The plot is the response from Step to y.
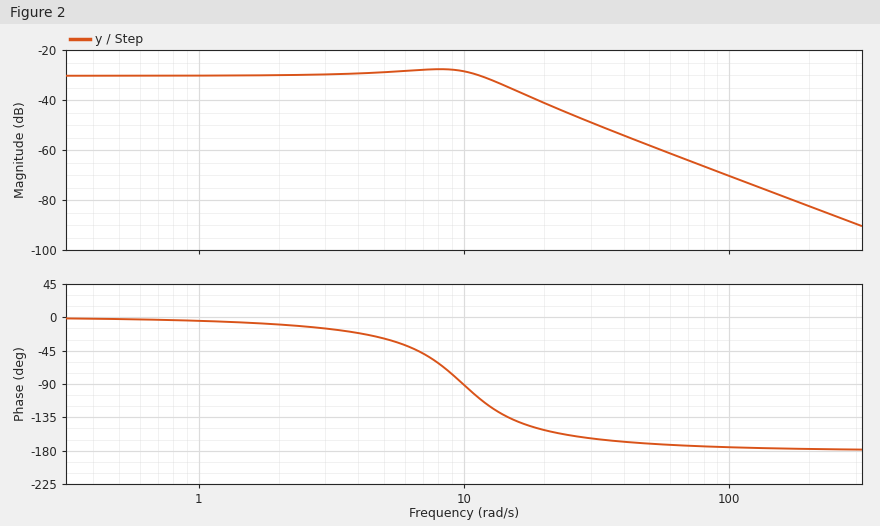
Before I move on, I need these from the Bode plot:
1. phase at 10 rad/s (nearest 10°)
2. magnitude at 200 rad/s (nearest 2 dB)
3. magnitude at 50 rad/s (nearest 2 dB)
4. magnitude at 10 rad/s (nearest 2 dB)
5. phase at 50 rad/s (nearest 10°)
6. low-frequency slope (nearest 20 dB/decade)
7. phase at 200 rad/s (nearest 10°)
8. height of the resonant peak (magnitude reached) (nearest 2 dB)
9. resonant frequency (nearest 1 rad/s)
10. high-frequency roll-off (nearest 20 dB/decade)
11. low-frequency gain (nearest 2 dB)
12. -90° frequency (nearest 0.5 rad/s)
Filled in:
-90°
-82 dB
-58 dB
-28 dB
-170°
0 dB/decade
-180°
-28 dB
8 rad/s
-40 dB/decade
-30 dB
10.0 rad/s
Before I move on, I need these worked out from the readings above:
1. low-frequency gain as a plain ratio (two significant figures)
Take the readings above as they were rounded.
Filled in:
0.032
